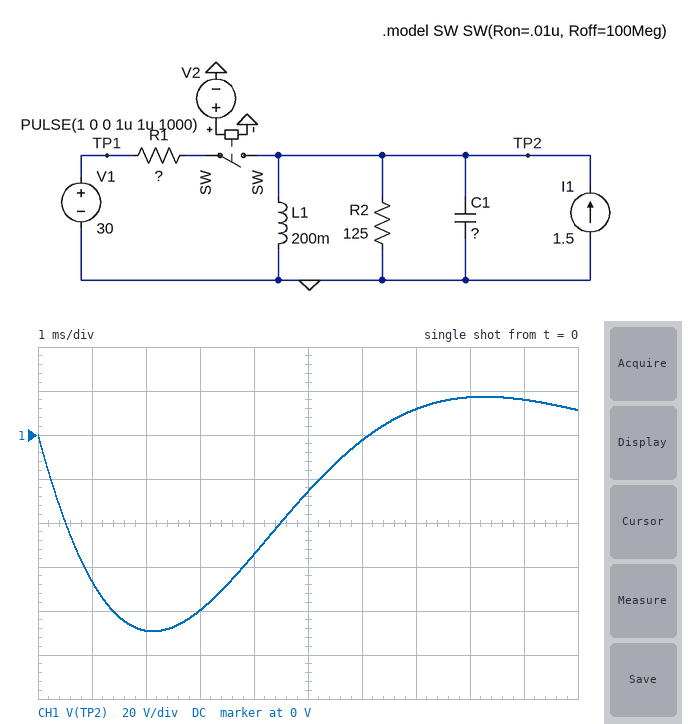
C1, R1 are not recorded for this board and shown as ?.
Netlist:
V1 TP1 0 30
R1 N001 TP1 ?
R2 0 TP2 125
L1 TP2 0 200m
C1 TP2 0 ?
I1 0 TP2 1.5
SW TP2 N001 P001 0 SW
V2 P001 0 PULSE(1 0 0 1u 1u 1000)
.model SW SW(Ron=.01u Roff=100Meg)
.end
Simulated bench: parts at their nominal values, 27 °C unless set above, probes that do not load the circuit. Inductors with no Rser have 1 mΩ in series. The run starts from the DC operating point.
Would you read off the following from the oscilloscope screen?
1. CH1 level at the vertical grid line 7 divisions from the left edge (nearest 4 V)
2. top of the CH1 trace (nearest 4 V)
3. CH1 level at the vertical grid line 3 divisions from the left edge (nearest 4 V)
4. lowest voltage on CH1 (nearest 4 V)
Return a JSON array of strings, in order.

["12 V", "16 V", "-80 V", "-88 V"]
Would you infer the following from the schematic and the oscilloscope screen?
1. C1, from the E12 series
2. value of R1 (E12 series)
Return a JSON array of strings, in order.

["15 µF", "22 Ω"]
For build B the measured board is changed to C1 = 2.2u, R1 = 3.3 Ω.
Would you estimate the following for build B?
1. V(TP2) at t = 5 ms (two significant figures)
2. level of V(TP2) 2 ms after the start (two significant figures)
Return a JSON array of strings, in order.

["-37 V", "-400 V"]
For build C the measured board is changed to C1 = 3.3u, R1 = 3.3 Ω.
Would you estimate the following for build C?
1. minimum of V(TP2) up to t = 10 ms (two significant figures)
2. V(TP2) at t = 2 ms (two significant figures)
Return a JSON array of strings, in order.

["-830 V", "-470 V"]
